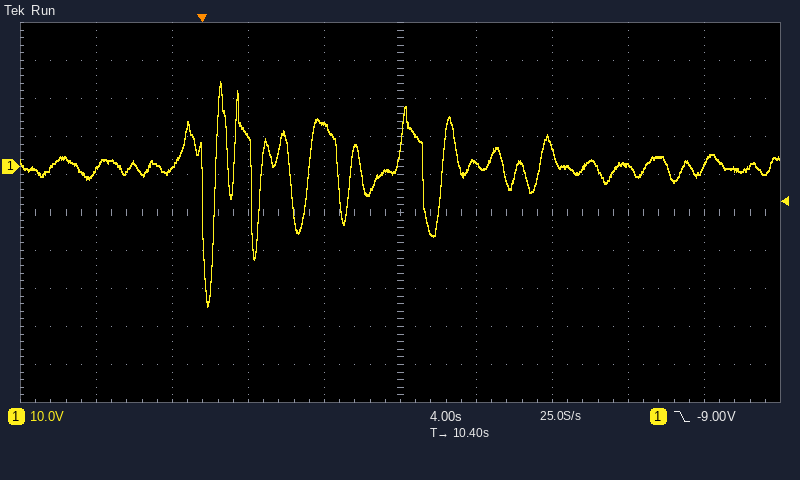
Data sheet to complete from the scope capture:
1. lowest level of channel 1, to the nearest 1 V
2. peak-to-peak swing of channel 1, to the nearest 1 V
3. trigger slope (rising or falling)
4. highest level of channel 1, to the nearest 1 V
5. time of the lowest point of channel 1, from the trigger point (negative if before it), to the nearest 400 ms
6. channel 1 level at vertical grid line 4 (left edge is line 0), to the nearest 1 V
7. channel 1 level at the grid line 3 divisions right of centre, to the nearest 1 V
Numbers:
-37 V
59 V
falling
22 V
+400 ms
11 V
0 V
